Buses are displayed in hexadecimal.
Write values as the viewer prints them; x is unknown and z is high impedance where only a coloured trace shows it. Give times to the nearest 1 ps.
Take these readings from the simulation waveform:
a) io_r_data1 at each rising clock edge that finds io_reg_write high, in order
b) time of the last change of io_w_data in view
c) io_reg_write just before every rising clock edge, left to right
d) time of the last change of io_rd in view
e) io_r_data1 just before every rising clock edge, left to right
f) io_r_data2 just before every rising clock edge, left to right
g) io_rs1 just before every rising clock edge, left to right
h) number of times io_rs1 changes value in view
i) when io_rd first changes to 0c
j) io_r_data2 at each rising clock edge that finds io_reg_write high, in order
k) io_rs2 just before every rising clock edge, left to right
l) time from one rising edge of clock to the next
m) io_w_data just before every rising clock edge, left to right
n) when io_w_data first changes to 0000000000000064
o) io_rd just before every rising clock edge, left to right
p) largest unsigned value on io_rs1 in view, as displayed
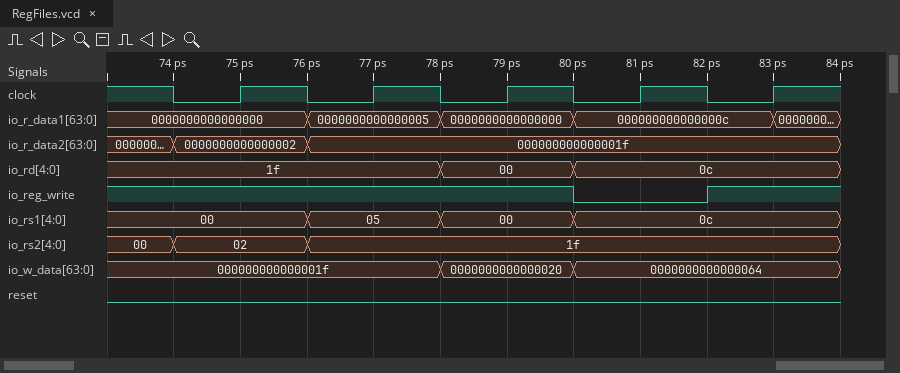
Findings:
0000000000000000, 0000000000000005, 0000000000000000, 000000000000000c
80 ps
1 1 1 0 1
80 ps
0000000000000000, 0000000000000005, 0000000000000000, 000000000000000c, 000000000000000c
0000000000000002, 000000000000001f, 000000000000001f, 000000000000001f, 000000000000001f
00, 05, 00, 0c, 0c
3
80 ps
0000000000000002, 000000000000001f, 000000000000001f, 000000000000001f
02, 1f, 1f, 1f, 1f
2 ps
000000000000001f, 000000000000001f, 0000000000000020, 0000000000000064, 0000000000000064
80 ps
1f, 1f, 00, 0c, 0c
0c
